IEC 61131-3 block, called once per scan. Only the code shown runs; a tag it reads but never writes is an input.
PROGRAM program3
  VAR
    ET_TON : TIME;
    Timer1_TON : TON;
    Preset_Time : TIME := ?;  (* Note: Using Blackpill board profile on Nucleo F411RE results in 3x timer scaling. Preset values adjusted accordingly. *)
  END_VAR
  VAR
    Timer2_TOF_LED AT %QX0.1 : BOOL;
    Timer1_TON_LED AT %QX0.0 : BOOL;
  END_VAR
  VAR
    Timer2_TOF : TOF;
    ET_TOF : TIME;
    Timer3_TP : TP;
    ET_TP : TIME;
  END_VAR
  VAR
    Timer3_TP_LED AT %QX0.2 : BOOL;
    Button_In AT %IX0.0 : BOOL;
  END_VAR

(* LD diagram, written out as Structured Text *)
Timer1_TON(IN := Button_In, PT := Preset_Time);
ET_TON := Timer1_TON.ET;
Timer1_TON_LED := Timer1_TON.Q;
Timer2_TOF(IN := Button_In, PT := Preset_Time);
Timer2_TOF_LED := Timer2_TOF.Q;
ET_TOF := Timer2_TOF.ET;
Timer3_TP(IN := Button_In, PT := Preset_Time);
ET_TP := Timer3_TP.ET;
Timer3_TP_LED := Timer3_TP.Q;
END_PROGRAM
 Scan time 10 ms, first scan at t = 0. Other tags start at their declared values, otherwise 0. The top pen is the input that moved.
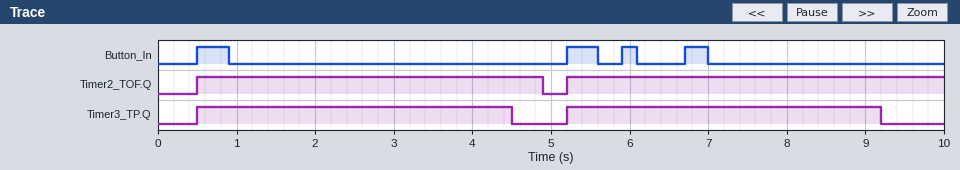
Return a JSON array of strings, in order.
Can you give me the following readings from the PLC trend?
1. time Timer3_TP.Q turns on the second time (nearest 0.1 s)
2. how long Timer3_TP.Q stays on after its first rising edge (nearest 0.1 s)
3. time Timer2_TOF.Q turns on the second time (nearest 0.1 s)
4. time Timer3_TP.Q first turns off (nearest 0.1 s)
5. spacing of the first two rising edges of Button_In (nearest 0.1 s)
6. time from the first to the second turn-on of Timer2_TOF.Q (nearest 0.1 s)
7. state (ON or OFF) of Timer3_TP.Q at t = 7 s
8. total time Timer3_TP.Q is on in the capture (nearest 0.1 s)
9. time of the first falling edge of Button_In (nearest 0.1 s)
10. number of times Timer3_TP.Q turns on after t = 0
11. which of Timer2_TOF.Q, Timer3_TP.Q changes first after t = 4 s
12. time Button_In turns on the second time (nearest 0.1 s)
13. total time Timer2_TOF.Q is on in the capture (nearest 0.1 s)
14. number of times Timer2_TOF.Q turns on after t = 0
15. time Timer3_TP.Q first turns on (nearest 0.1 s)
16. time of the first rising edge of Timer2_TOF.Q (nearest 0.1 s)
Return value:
["5.2 s", "4.0 s", "5.2 s", "4.5 s", "4.7 s", "4.7 s", "ON", "8.0 s", "0.9 s", "2", "Timer3_TP.Q", "5.2 s", "9.2 s", "2", "0.5 s", "0.5 s"]
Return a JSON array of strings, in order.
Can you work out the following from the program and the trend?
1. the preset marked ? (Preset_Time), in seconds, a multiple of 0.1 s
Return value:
["4.0 s"]
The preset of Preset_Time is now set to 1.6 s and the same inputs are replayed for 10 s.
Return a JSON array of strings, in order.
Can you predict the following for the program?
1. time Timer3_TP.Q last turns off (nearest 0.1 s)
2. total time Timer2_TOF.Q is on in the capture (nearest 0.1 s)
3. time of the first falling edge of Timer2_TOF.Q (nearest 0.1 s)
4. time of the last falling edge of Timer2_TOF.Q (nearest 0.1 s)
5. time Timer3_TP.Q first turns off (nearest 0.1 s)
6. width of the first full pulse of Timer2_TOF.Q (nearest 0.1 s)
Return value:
["6.8 s", "5.4 s", "2.5 s", "8.6 s", "2.1 s", "2.0 s"]
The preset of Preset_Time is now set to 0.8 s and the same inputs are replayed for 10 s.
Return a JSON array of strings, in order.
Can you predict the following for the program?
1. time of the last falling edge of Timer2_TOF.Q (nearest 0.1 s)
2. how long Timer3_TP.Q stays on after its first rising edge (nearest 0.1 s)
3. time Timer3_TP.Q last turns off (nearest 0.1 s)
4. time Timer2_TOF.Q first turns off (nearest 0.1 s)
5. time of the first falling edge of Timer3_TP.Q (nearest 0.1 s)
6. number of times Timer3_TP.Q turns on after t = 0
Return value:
["7.8 s", "0.8 s", "7.5 s", "1.7 s", "1.3 s", "3"]
